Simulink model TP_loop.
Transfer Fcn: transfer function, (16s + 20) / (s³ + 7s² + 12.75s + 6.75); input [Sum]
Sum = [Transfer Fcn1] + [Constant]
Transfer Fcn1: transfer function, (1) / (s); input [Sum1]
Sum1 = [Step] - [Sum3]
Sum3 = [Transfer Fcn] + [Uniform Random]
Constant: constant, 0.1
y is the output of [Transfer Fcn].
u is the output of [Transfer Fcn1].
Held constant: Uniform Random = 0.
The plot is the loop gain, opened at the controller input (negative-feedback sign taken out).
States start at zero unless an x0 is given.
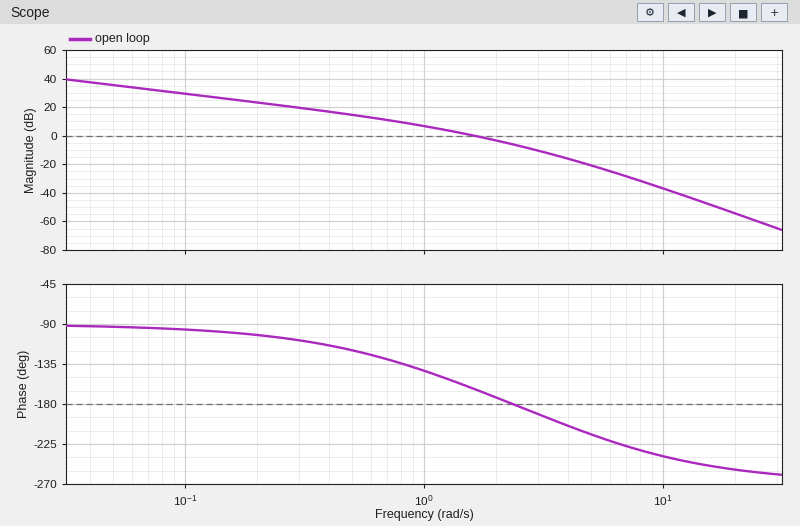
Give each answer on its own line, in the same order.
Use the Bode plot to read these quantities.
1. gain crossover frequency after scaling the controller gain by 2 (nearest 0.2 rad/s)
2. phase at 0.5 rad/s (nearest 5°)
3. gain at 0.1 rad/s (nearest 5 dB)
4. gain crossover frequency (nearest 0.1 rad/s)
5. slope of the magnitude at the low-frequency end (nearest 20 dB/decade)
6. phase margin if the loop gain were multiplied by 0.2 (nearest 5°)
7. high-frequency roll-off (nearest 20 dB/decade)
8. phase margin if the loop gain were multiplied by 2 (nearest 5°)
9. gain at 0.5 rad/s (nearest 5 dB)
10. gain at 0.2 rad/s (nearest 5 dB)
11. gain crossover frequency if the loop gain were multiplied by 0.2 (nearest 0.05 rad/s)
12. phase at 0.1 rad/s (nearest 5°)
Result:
2.4 rad/s
-120°
30 dB
1.6 rad/s
-20 dB/decade
60°
-60 dB/decade
0°
15 dB
25 dB
0.55 rad/s
-95°
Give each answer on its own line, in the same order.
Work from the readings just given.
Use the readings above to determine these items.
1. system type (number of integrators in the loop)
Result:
1
